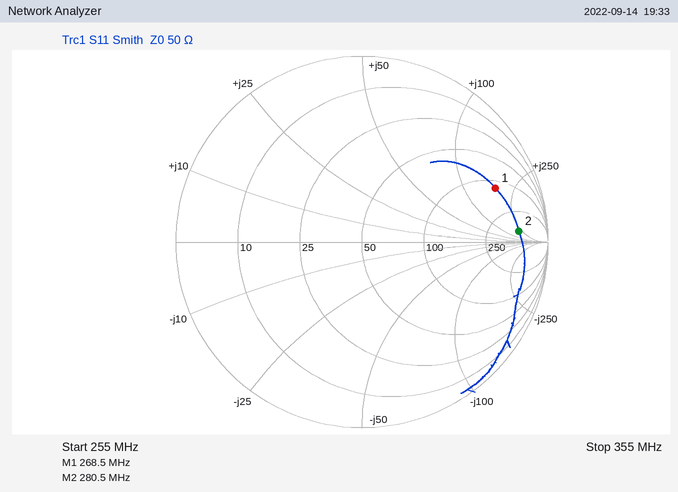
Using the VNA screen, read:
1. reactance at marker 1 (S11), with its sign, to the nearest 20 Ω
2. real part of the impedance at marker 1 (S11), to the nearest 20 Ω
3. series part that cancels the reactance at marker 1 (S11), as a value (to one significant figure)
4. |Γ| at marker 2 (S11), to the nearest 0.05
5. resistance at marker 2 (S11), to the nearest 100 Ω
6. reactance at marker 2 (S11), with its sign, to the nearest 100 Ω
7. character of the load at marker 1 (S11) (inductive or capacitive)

+180 Ω
120 Ω
3 pF
0.85
500 Ω
+200 Ω
inductive
